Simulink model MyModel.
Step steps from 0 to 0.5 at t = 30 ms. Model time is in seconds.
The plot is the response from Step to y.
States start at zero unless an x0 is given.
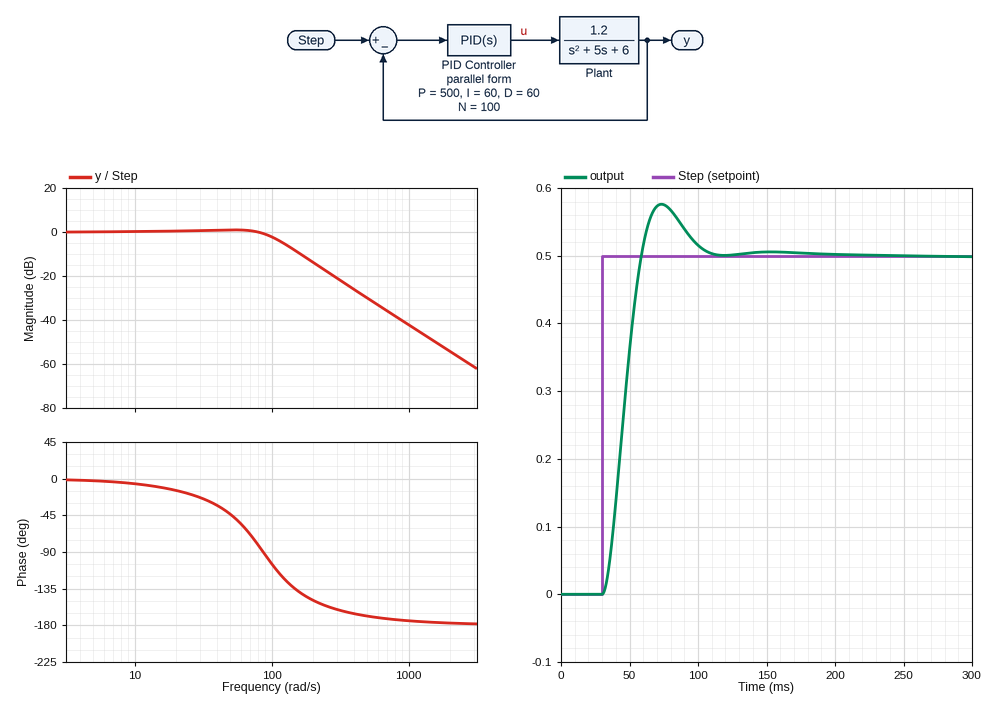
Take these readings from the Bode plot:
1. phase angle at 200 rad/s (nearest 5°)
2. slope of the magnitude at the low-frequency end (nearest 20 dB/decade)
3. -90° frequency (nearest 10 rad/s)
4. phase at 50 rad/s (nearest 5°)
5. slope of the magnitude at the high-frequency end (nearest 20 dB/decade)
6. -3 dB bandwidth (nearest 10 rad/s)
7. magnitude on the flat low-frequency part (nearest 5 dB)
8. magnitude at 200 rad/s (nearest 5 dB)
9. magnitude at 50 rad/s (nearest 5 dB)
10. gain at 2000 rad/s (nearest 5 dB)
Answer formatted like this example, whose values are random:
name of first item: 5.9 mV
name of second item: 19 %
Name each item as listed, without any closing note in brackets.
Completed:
phase angle at 200 rad/s: -150°
slope of the magnitude at the low-frequency end: 0 dB/decade
-90° frequency: 90 rad/s
phase at 50 rad/s: -45°
slope of the magnitude at the high-frequency end: -40 dB/decade
-3 dB bandwidth: 110 rad/s
magnitude on the flat low-frequency part: 0 dB
magnitude at 200 rad/s: -15 dB
magnitude at 50 rad/s: 0 dB
gain at 2000 rad/s: -55 dB
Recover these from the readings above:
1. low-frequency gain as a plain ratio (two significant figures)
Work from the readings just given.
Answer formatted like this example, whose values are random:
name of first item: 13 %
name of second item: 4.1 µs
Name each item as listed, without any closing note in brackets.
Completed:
low-frequency gain as a plain ratio: 1.0
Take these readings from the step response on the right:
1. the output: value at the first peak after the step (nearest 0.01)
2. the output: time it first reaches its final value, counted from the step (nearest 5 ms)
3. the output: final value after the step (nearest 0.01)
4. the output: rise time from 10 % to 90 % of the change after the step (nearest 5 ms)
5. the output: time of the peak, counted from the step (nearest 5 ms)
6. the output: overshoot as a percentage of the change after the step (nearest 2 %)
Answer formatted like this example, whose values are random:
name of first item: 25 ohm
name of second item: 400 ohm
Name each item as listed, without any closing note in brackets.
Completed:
the output: value at the first peak after the step: 0.58
the output: time it first reaches its final value, counted from the step: 30 ms
the output: final value after the step: 0.50
the output: rise time from 10 % to 90 % of the change after the step: 20 ms
the output: time of the peak, counted from the step: 45 ms
the output: overshoot as a percentage of the change after the step: 16 %
